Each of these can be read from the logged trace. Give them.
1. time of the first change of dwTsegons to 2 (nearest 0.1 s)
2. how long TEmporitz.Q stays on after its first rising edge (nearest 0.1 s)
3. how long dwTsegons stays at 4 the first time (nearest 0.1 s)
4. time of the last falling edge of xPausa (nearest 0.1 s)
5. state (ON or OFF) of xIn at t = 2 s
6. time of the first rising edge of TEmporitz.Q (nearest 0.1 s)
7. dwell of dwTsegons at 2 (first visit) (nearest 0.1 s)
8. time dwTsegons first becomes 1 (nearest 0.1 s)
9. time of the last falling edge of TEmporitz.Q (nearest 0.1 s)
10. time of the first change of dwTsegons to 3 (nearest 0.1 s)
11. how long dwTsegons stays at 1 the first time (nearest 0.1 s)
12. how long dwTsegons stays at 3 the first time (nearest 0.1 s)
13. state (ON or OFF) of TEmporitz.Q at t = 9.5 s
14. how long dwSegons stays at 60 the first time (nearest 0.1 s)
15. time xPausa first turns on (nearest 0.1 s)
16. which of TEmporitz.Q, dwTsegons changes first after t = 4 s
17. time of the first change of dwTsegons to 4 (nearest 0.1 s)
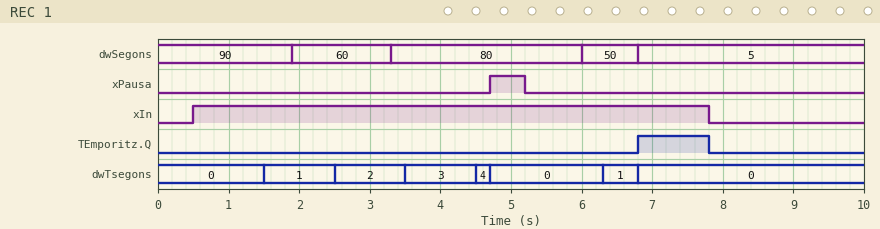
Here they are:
2.5 s
1.0 s
0.2 s
5.2 s
ON
6.8 s
1.0 s
1.5 s
7.8 s
3.5 s
1.0 s
1.0 s
OFF
1.4 s
4.7 s
dwTsegons
4.5 s
